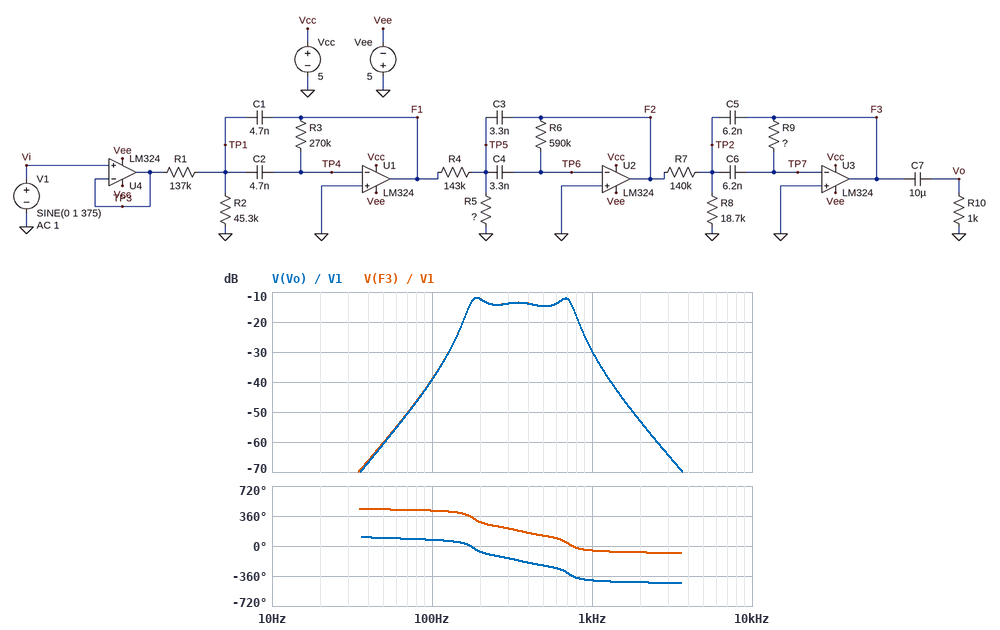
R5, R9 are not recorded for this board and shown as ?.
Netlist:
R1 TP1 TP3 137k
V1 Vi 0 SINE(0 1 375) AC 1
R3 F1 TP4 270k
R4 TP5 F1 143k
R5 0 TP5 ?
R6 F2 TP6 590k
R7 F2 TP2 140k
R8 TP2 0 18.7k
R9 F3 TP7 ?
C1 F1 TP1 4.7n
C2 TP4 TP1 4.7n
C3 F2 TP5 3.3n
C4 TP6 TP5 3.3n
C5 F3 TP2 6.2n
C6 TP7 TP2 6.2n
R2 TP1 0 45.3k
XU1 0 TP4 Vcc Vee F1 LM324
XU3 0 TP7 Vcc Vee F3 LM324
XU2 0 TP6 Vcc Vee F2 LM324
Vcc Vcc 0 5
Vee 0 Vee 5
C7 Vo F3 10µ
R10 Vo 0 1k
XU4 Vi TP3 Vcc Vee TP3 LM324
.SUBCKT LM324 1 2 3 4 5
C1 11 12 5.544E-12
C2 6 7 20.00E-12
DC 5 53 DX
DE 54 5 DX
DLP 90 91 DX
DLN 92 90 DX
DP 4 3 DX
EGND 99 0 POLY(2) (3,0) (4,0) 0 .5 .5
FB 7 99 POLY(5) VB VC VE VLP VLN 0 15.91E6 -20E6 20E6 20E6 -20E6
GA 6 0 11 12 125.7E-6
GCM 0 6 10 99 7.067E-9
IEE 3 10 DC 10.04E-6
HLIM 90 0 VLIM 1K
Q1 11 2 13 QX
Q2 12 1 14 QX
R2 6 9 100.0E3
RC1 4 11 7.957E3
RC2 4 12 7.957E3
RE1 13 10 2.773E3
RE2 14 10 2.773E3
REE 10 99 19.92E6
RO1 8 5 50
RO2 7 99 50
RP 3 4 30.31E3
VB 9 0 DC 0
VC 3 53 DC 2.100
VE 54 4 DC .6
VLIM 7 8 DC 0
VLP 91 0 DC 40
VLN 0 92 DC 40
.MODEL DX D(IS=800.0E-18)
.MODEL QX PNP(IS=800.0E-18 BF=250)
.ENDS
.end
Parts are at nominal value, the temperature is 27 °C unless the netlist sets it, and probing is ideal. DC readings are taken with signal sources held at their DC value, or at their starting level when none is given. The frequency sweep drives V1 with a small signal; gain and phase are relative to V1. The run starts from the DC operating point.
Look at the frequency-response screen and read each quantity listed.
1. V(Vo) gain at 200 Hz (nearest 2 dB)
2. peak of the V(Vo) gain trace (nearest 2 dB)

-12 dB
-12 dB
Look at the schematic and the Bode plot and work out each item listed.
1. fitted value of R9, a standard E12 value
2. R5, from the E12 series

1.2 MΩ
8.2 kΩ
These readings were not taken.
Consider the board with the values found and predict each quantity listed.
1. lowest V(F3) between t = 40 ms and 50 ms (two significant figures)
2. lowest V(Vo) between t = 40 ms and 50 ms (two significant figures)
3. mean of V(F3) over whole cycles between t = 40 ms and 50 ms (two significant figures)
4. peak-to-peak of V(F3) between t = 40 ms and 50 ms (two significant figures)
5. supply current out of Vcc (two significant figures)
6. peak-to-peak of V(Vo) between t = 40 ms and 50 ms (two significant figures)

-230 mV
-210 mV
-24 mV
420 mV
1.4 mA
420 mV
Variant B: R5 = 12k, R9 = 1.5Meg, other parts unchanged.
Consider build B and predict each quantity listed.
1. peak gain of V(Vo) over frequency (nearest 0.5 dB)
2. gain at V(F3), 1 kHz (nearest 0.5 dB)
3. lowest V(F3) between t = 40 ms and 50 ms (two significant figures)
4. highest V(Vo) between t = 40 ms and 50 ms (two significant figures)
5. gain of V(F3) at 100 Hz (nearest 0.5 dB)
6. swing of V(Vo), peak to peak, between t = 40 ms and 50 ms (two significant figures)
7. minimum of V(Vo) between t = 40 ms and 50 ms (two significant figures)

-8.0 dB
-32.0 dB
-360 mV
330 mV
-33.0 dB
660 mV
-330 mV
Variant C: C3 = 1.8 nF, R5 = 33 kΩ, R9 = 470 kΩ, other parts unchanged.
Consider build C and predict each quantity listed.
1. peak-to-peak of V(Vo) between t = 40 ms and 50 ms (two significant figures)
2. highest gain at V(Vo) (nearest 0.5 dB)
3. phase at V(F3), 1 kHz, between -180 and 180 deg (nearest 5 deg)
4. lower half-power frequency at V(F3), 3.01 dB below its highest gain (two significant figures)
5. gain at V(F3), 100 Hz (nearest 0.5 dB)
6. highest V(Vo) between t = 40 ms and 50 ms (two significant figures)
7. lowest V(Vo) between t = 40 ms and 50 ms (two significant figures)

2.9 V
4.0 dB
-50 deg
280 Hz
-38.5 dB
1.4 V
-1.4 V
